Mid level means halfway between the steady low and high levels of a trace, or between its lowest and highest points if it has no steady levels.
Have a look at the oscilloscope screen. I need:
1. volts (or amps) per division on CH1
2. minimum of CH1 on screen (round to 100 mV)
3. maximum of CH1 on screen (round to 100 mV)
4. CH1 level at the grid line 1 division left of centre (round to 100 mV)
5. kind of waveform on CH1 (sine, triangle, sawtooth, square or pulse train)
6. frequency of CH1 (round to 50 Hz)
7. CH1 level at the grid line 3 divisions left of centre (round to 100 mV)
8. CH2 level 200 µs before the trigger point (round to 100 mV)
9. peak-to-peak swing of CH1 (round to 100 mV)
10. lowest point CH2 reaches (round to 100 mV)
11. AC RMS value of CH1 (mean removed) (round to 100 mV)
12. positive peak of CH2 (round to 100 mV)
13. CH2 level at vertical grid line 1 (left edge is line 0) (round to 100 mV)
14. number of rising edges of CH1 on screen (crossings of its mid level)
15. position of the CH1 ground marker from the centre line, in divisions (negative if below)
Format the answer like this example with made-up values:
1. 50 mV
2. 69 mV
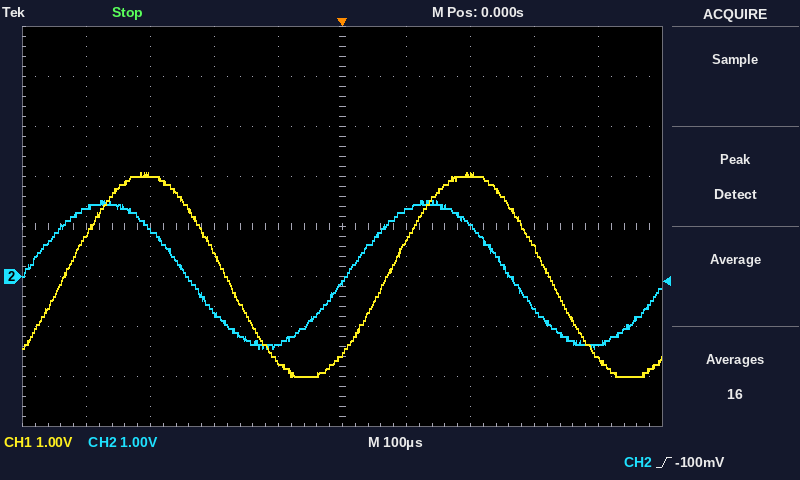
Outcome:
1. 1 V
2. -2.0 V
3. 2.1 V
4. -1.7 V
5. sine
6. 2.00 kHz
7. 2.0 V
8. -700 mV
9. 4.1 V
10. -1.4 V
11. 1.4 V
12. 1.5 V
13. 1.4 V
14. 2
15. -1.0 div
